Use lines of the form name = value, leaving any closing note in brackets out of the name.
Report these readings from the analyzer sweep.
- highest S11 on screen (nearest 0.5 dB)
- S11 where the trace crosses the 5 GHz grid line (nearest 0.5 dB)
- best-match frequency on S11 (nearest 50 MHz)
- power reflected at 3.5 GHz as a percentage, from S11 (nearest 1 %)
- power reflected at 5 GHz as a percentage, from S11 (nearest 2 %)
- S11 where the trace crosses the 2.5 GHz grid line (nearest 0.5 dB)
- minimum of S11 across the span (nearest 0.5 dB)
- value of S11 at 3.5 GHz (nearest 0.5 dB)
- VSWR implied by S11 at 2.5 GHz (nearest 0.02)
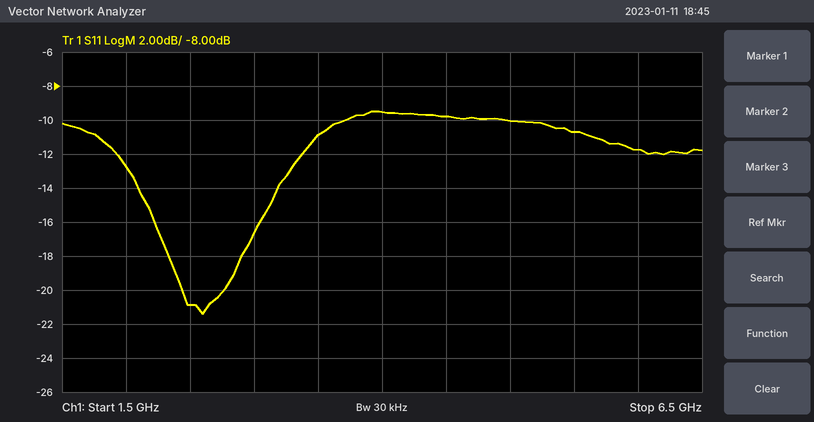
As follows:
highest S11 on screen = -9.5 dB
S11 where the trace crosses the 5 GHz grid line = -10.0 dB
best-match frequency on S11 = 2.60 GHz
power reflected at 3.5 GHz as a percentage, from S11 = 8 %
power reflected at 5 GHz as a percentage, from S11 = 10 %
S11 where the trace crosses the 2.5 GHz grid line = -21.0 dB
minimum of S11 across the span = -21.5 dB
value of S11 at 3.5 GHz = -11.0 dB
VSWR implied by S11 at 2.5 GHz = 1.20
